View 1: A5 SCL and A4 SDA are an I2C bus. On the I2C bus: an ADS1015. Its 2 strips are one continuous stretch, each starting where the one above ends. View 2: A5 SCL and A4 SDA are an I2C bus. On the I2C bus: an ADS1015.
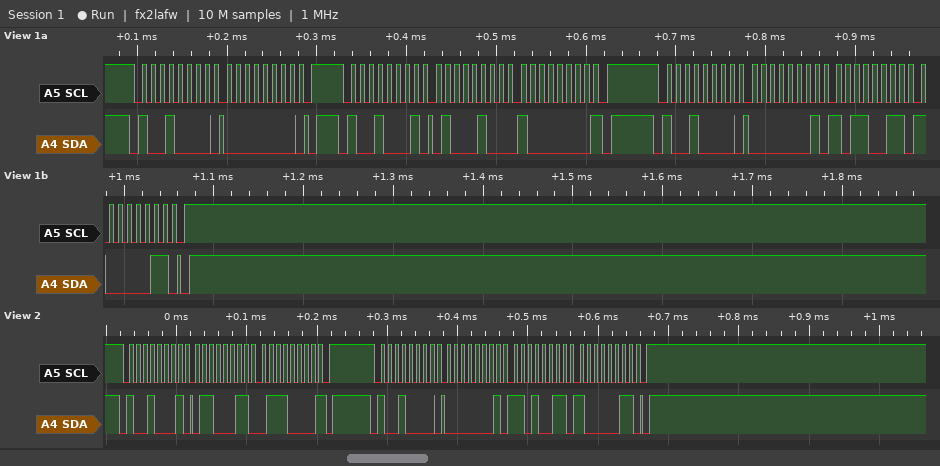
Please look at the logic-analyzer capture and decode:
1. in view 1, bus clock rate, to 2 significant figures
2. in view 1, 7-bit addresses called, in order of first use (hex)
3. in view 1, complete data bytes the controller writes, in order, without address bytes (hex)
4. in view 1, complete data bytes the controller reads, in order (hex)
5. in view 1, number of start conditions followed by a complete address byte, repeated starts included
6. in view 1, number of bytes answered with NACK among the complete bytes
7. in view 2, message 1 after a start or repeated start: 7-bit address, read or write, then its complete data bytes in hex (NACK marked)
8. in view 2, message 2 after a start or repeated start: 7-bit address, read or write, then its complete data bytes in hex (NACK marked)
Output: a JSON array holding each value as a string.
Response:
["100 kHz", "0x48", "00 01 B3 83", "44 80", "3", "1", "0x48 read: 63 70 NACK", "0x48 write: 01 D3 83"]
